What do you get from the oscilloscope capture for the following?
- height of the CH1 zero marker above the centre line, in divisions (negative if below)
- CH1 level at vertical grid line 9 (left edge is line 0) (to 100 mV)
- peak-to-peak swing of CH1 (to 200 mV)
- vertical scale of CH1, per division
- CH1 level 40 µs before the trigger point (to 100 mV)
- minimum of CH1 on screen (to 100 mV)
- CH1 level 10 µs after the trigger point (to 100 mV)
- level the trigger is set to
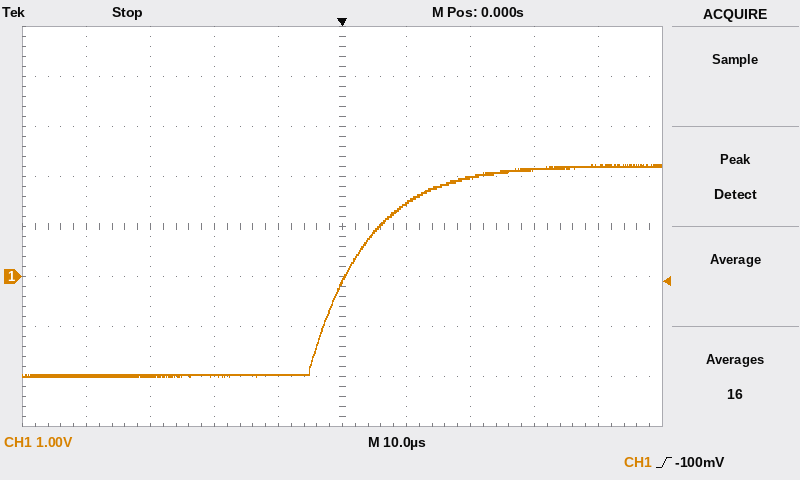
-1.0 div
2.2 V
4.2 V
1 V
-2.0 V
-2.0 V
1.5 V
-100 mV
